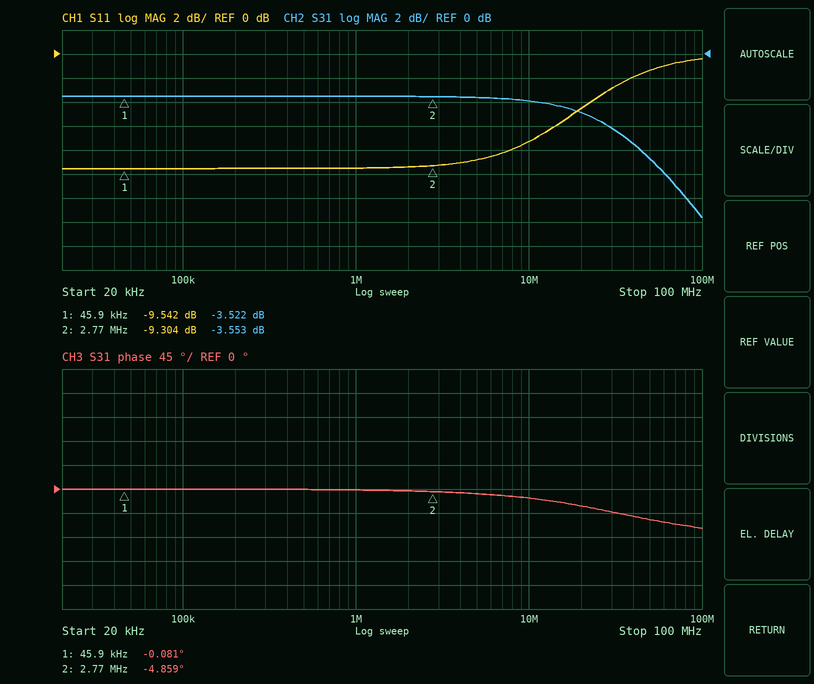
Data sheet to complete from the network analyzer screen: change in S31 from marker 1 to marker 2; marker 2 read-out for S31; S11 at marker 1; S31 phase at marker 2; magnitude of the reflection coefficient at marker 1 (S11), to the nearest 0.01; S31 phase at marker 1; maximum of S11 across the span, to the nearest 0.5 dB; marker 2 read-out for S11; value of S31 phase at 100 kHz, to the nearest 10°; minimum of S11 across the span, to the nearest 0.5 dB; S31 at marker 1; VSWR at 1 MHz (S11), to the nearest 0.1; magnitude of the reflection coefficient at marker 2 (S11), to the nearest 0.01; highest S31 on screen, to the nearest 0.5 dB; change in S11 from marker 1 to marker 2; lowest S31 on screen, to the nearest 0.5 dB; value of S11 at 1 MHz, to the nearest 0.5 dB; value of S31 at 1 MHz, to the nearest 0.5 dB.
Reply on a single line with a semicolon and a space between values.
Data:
-0.031 dB; -3.553 dB; -9.542 dB; -4.859°; 0.33; -0.081°; -0.5 dB; -9.304 dB; 0°; -9.5 dB; -3.522 dB; 2.0; 0.34; -3.5 dB; 0.238 dB; -13.5 dB; -9.5 dB; -3.5 dB
